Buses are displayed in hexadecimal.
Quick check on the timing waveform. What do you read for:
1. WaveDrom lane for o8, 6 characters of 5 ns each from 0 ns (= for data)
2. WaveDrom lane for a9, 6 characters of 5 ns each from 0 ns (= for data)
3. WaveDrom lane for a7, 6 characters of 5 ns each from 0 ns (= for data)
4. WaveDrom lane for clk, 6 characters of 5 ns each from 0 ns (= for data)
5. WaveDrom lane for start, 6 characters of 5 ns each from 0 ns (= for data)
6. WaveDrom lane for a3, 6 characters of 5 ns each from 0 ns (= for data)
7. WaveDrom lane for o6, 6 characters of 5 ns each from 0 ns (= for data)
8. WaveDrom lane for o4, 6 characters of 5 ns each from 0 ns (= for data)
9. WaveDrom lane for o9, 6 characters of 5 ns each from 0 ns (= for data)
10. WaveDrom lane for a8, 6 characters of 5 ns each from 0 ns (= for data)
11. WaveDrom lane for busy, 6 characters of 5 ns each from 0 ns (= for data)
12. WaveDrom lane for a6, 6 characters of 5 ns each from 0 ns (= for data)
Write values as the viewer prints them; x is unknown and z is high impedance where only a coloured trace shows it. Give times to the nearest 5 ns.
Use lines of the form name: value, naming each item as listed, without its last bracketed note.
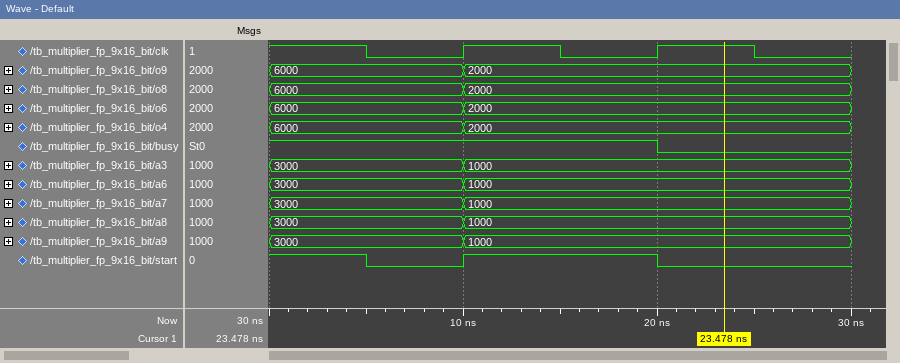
WaveDrom lane for o8, 6 characters of 5 ns each from 0 ns: {name: 'o8', wave: '=.=...', data: '6000 2000'}
WaveDrom lane for a9, 6 characters of 5 ns each from 0 ns: {name: 'a9', wave: '=.=...', data: '3000 1000'}
WaveDrom lane for a7, 6 characters of 5 ns each from 0 ns: {name: 'a7', wave: '=.=...', data: '3000 1000'}
WaveDrom lane for clk, 6 characters of 5 ns each from 0 ns: {name: 'clk', wave: '101010'}
WaveDrom lane for start, 6 characters of 5 ns each from 0 ns: {name: 'start', wave: '101.0.'}
WaveDrom lane for a3, 6 characters of 5 ns each from 0 ns: {name: 'a3', wave: '=.=...', data: '3000 1000'}
WaveDrom lane for o6, 6 characters of 5 ns each from 0 ns: {name: 'o6', wave: '=.=...', data: '6000 2000'}
WaveDrom lane for o4, 6 characters of 5 ns each from 0 ns: {name: 'o4', wave: '=.=...', data: '6000 2000'}
WaveDrom lane for o9, 6 characters of 5 ns each from 0 ns: {name: 'o9', wave: '=.=...', data: '6000 2000'}
WaveDrom lane for a8, 6 characters of 5 ns each from 0 ns: {name: 'a8', wave: '=.=...', data: '3000 1000'}
WaveDrom lane for busy, 6 characters of 5 ns each from 0 ns: {name: 'busy', wave: '1...0.'}
WaveDrom lane for a6, 6 characters of 5 ns each from 0 ns: {name: 'a6', wave: '=.=...', data: '3000 1000'}
